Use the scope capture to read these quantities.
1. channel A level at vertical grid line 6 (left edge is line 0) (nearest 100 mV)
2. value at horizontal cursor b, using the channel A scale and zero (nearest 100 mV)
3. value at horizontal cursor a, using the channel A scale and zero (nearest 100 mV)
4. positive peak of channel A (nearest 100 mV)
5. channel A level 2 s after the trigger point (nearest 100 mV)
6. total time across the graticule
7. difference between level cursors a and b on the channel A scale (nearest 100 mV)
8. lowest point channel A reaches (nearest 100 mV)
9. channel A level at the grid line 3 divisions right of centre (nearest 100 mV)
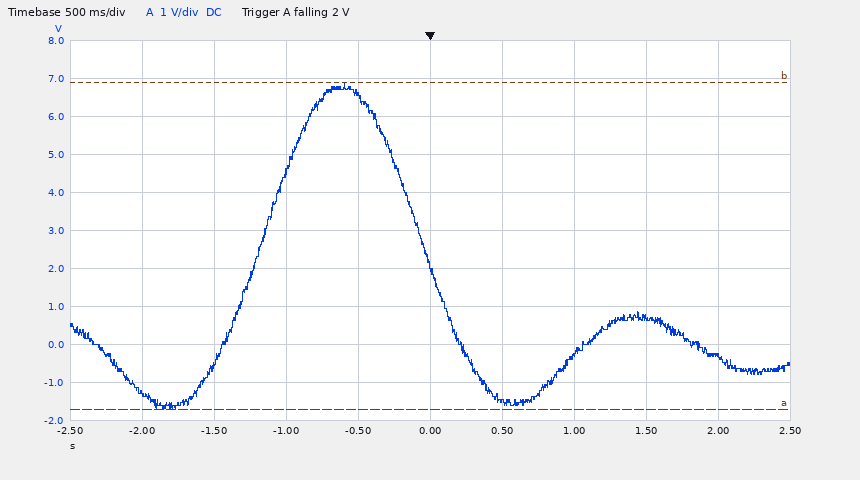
-1.5 V
6.9 V
-1.7 V
6.9 V
-300 mV
5 s
8.6 V
-1.7 V
700 mV
